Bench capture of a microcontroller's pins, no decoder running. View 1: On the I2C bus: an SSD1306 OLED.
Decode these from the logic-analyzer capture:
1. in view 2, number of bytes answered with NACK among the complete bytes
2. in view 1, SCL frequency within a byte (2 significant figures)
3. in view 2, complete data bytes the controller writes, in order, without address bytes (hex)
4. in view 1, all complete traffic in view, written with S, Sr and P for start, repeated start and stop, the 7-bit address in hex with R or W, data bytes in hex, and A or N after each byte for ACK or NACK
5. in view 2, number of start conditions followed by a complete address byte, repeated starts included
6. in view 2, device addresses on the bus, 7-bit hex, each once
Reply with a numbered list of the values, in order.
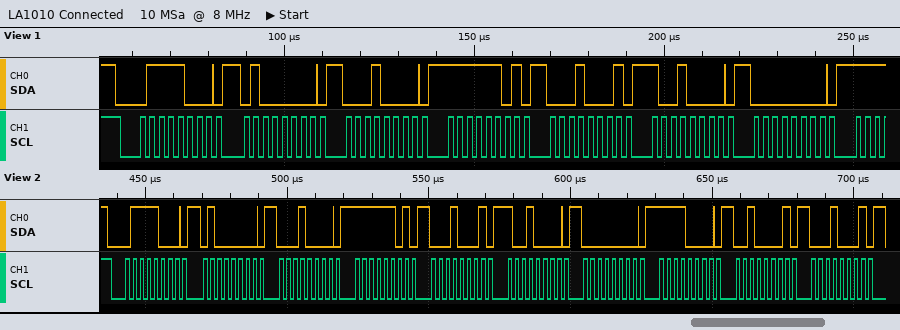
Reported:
1. 0
2. 400 kHz
3. 40 10 FD 11 90 00 F0 21 11
4. S 3CW A 40 A 10 A FD A 11 A 90 A 00 A
5. 1
6. 0x3C
